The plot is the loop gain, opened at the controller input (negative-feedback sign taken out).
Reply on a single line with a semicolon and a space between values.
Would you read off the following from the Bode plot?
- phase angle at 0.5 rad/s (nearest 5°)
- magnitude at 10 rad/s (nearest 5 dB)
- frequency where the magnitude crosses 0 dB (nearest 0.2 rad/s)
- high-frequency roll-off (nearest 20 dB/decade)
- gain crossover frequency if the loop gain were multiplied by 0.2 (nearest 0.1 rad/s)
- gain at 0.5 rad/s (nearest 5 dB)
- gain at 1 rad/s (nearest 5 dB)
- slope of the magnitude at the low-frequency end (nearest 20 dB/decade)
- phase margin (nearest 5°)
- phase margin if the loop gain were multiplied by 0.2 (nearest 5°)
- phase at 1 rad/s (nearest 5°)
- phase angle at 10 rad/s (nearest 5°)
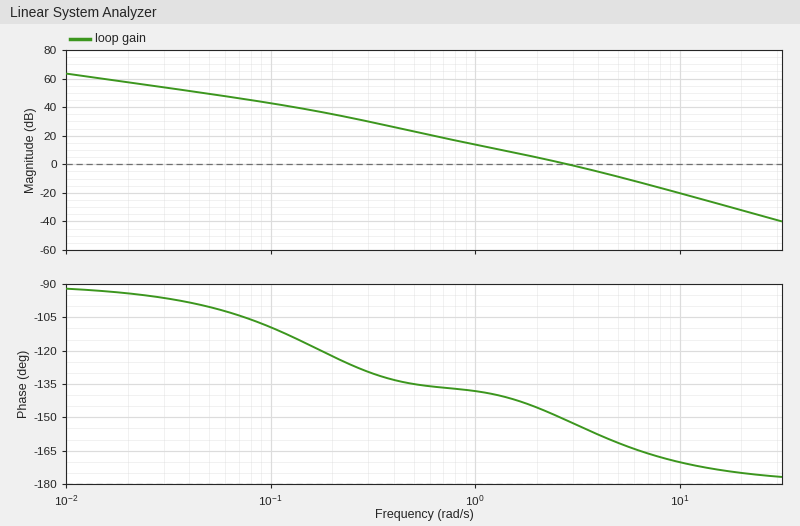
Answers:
-135°; -20 dB; 2.8 rad/s; -40 dB/decade; 1.0 rad/s; 25 dB; 15 dB; -20 dB/decade; 30°; 40°; -140°; -170°
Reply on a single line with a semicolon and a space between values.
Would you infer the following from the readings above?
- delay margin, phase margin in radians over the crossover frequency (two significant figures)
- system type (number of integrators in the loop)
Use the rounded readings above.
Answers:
0.19 s; 1
